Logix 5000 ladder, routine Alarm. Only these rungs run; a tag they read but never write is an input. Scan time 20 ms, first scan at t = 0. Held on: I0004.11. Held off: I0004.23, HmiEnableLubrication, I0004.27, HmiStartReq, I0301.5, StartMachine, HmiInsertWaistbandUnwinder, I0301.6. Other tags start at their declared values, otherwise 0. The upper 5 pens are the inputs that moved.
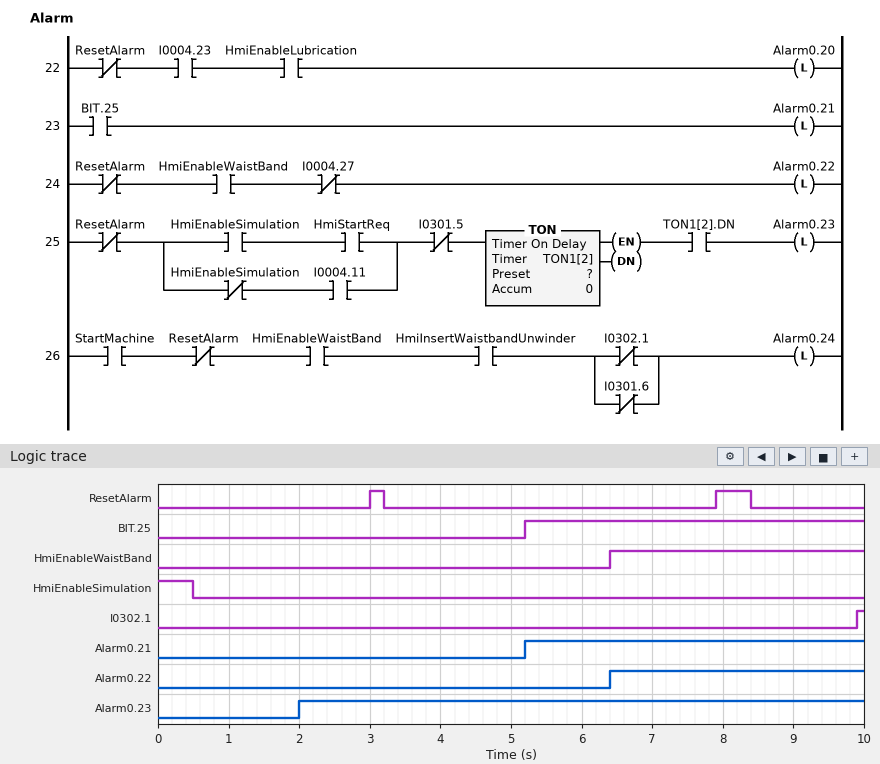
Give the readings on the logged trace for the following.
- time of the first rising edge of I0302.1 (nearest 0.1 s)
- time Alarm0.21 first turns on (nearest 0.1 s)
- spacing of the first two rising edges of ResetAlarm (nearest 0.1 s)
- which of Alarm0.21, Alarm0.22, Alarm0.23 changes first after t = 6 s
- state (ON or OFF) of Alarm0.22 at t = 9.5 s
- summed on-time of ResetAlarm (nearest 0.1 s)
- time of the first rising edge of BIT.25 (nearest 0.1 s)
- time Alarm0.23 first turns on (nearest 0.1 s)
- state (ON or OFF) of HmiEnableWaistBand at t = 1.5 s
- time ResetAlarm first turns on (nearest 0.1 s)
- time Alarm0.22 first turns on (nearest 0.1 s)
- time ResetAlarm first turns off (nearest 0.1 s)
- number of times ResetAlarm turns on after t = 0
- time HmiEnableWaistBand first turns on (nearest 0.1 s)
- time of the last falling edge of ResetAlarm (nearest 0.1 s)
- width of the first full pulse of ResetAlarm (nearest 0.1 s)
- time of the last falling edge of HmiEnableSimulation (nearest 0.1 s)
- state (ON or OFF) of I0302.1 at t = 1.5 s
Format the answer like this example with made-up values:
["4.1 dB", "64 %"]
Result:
["9.9 s", "5.2 s", "4.9 s", "Alarm0.22", "ON", "0.7 s", "5.2 s", "2.0 s", "OFF", "3.0 s", "6.4 s", "3.2 s", "2", "6.4 s", "8.4 s", "0.2 s", "0.5 s", "OFF"]
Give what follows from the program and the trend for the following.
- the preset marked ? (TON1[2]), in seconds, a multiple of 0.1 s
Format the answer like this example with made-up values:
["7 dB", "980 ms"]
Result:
["1.5 s"]
